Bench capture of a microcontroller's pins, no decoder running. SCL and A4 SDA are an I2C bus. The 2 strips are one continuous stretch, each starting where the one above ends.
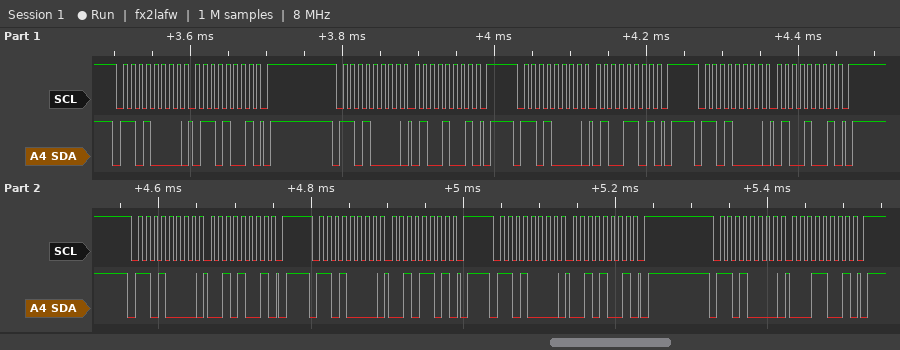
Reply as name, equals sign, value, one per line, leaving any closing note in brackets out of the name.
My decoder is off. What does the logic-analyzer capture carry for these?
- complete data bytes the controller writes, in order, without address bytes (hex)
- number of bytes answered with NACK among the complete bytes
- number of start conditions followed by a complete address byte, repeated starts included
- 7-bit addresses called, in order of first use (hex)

complete data bytes the controller writes, in order, without address bytes = 69 49 4D 49 29 2D 29 19
number of bytes answered with NACK among the complete bytes = 0
number of start conditions followed by a complete address byte, repeated starts included = 8
7-bit addresses called, in order of first use = 0x68
